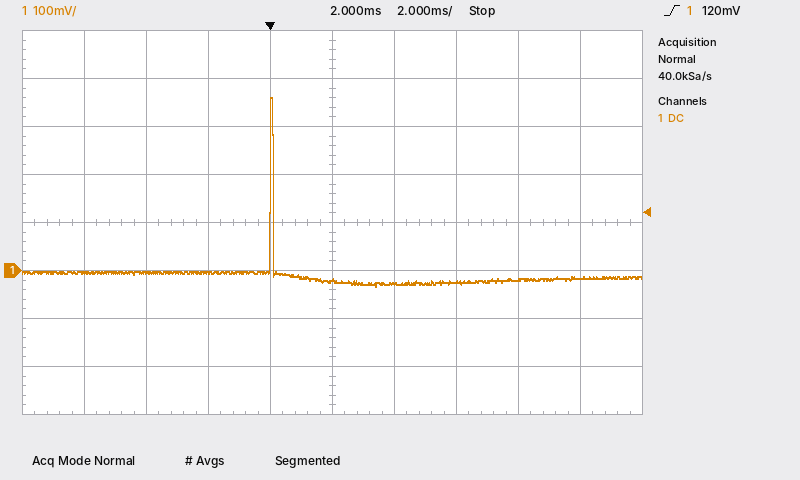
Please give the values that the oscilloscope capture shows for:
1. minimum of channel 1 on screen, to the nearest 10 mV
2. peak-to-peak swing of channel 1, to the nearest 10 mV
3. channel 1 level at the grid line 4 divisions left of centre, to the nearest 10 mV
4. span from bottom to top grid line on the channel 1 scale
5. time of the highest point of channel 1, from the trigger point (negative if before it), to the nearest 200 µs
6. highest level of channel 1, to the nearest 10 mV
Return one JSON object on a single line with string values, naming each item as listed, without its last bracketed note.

{"minimum of channel 1 on screen, to the nearest 10 mV": "-30 mV", "peak-to-peak swing of channel 1, to the nearest 10 mV": "390 mV", "channel 1 level at the grid line 4 divisions left of centre, to the nearest 10 mV": "0 mV", "span from bottom to top grid line on the channel 1 scale": "800 mV", "time of the highest point of channel 1, from the trigger point (negative if before it), to the nearest 200 µs": "0.0 ms", "highest level of channel 1, to the nearest 10 mV": "360 mV"}
